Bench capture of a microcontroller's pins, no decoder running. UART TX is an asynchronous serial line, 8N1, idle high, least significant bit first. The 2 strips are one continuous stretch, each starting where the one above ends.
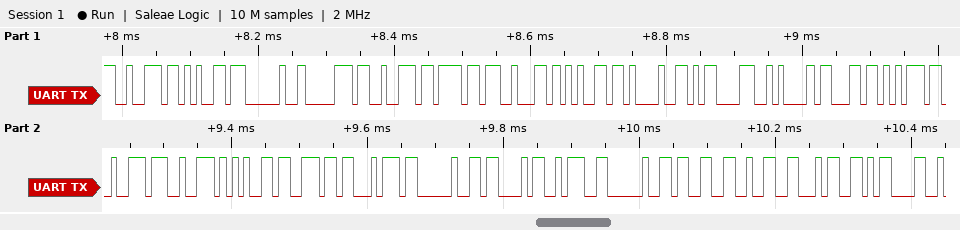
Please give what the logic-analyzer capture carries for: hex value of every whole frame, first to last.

72 65 20 70 72 6F 62 65 21 0D 0A 63 75 72 72 65 6E 74 20 43 3A 20 33 32 34 0D
